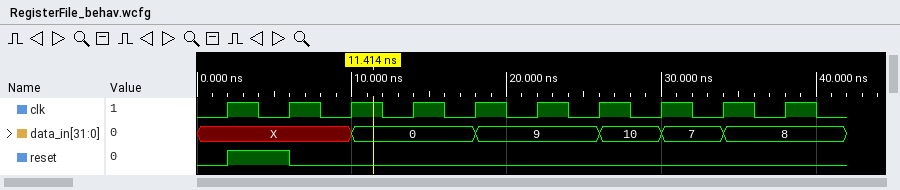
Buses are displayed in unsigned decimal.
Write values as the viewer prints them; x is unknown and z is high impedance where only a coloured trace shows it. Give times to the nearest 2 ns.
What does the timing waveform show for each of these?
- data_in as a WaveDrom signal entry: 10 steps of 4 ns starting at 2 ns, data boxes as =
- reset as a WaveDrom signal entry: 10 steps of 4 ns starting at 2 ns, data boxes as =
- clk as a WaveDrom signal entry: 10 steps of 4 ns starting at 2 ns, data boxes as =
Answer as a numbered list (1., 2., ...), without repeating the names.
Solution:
1. {name: 'data_in', wave: 'x.=.=.===.', data: '0 9 10 7 8'}
2. {name: 'reset', wave: '10........'}
3. {name: 'clk', wave: 'p.........'}
